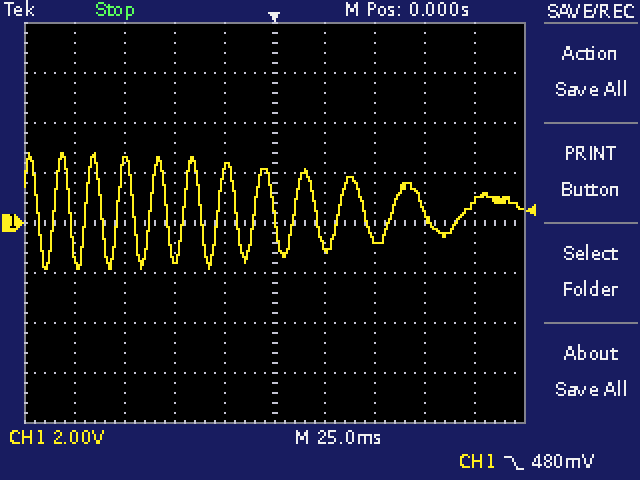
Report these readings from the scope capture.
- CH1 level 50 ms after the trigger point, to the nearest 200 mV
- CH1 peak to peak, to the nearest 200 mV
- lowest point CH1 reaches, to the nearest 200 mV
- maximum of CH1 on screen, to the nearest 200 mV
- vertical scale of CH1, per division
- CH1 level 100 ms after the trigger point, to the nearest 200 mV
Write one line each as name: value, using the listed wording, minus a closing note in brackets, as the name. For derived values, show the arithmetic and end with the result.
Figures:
CH1 level 50 ms after the trigger point, to the nearest 200 mV: -600 mV
CH1 peak to peak, to the nearest 200 mV: 2.8 V − (-1.8 V) = 4.6 V
lowest point CH1 reaches, to the nearest 200 mV: -1.8 V
maximum of CH1 on screen, to the nearest 200 mV: 2.8 V
vertical scale of CH1, per division: 2 V
CH1 level 100 ms after the trigger point, to the nearest 200 mV: 800 mV
